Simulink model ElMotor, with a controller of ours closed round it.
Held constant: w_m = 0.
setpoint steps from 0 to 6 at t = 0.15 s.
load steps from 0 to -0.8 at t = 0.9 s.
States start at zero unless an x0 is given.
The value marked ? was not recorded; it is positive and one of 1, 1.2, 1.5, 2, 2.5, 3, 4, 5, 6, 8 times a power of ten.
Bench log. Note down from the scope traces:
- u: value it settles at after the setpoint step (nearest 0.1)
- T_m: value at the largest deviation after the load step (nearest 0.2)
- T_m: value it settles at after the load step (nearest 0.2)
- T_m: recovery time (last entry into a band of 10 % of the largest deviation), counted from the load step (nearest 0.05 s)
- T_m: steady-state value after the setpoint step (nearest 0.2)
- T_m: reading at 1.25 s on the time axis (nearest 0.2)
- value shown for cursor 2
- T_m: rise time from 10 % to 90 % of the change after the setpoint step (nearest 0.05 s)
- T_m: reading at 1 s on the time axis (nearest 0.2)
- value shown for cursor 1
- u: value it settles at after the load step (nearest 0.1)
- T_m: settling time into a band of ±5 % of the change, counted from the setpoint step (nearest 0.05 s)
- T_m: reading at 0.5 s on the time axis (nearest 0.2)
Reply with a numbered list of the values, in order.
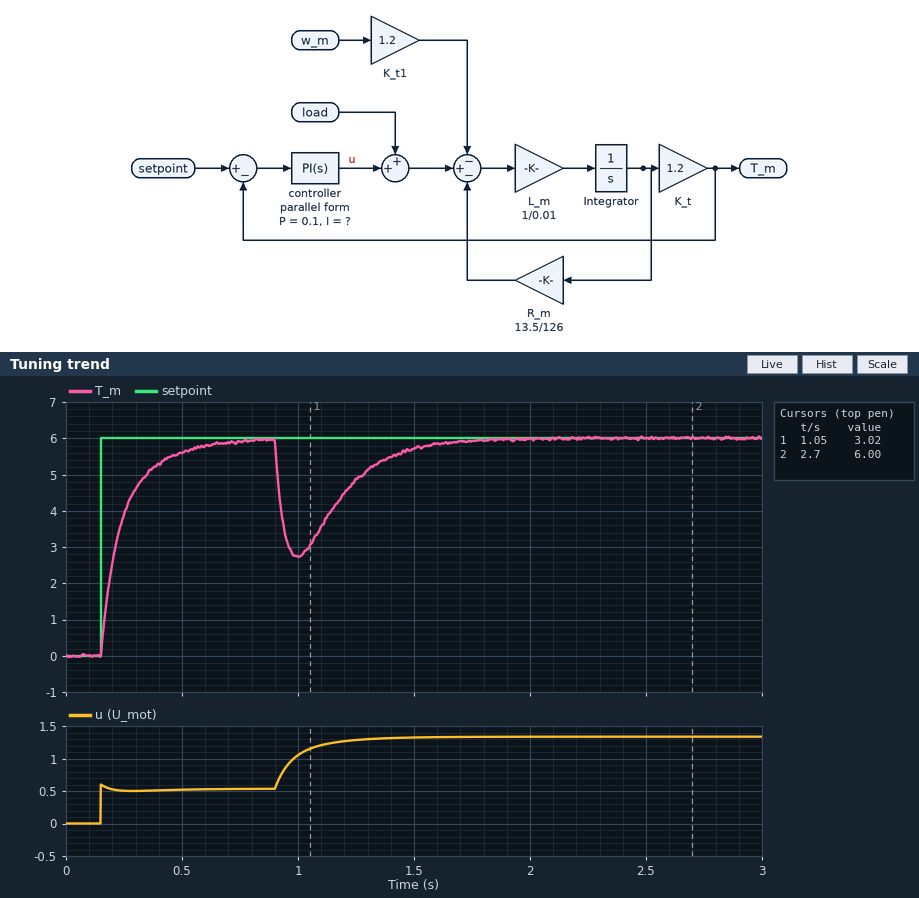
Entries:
1. 0.5
2. 2.8
3. 6.0
4. 0.60 s
5. 6.0
6. 4.8
7. 6.00
8. 0.25 s
9. 2.8
10. 3.02
11. 1.3
12. 0.40 s
13. 5.6
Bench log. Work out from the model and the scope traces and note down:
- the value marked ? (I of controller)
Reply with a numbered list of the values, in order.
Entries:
1. 0.8
